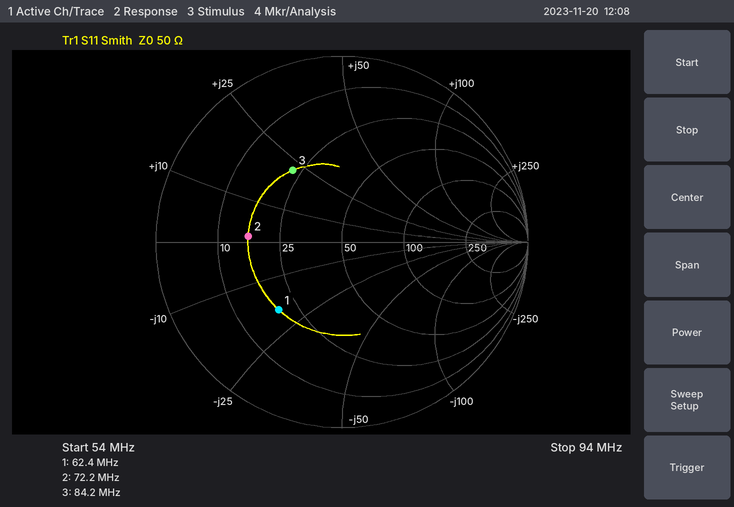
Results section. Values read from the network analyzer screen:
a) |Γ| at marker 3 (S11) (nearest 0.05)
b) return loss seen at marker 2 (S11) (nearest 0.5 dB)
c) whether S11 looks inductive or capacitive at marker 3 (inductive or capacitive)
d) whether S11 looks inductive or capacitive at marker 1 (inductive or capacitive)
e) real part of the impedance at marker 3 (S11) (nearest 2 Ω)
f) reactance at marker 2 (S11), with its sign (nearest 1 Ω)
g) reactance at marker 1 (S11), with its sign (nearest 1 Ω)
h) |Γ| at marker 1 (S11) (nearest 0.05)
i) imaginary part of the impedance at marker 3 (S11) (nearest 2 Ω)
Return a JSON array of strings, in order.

["0.45", "6.0 dB", "inductive", "capacitive", "22 Ω", "+1 Ω", "-19 Ω", "0.50", "+22 Ω"]
